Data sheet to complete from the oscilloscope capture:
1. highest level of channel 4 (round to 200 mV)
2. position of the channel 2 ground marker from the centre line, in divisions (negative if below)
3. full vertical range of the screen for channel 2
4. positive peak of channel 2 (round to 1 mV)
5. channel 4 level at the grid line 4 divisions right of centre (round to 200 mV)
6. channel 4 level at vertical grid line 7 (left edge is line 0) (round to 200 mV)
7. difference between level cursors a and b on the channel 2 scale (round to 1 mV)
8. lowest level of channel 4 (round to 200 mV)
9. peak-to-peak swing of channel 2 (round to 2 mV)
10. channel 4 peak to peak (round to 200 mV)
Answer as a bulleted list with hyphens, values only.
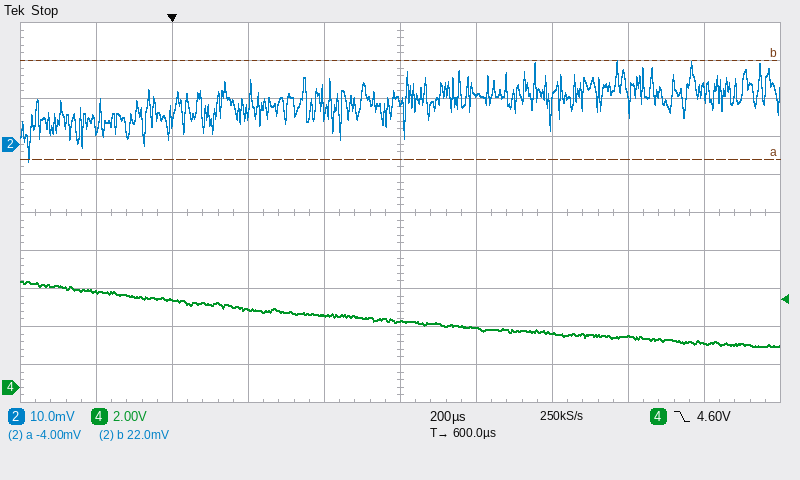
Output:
- 5.6 V
- +1.8 div
- 100 mV
- 22 mV
- 2.4 V
- 2.8 V
- 26 mV
- 2.2 V
- 26 mV
- 3.4 V
